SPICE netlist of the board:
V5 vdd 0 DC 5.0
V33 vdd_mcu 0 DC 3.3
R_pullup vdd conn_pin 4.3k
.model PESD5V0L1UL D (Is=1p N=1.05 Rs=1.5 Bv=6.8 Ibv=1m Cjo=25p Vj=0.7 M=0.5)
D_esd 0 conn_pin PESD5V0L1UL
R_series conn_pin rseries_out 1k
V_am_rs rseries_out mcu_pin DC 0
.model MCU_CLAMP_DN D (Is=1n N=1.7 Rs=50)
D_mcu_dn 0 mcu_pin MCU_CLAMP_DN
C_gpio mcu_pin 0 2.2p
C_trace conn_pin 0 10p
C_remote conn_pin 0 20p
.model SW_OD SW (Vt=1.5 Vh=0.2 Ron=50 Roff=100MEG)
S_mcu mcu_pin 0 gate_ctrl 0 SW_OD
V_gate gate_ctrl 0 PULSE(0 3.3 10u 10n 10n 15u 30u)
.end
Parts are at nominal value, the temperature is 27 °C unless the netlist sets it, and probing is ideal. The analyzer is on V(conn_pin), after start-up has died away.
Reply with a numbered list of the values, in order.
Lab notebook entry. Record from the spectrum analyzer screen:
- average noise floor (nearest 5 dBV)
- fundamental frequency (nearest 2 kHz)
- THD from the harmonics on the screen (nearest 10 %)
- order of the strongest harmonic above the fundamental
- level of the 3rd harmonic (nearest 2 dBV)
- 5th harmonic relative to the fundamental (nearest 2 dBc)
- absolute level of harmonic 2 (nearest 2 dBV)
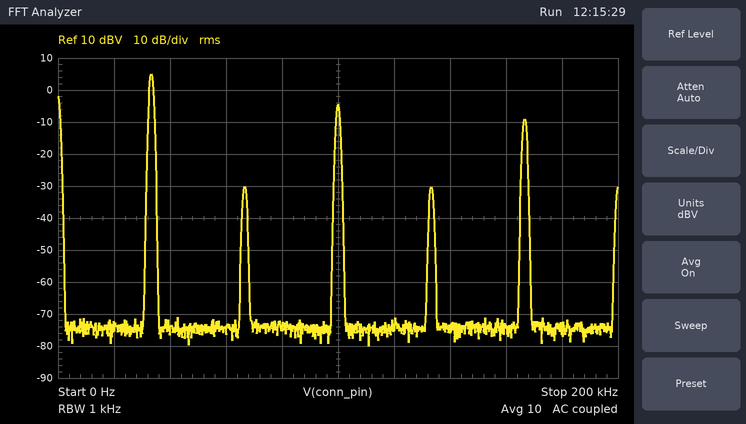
1. -75 dBV
2. 34 kHz
3. 40 %
4. 3
5. -4 dBV
6. -14 dBc
7. -30 dBV
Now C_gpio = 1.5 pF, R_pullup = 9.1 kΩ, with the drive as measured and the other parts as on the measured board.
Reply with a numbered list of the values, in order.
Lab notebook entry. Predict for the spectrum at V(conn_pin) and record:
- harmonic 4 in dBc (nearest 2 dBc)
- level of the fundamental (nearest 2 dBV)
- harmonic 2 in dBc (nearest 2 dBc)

1. -28 dBc
2. 6 dBV
3. -28 dBc
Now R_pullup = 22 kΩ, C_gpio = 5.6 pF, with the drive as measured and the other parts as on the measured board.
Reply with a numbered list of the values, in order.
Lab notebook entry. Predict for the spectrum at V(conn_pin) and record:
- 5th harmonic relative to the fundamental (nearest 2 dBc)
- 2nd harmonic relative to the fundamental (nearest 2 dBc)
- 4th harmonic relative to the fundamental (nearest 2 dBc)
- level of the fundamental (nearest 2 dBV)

1. -16 dBc
2. -20 dBc
3. -22 dBc
4. 6 dBV
